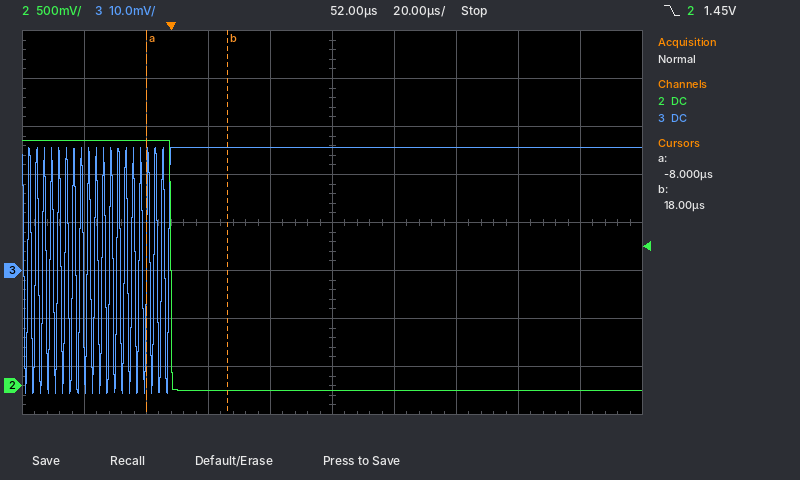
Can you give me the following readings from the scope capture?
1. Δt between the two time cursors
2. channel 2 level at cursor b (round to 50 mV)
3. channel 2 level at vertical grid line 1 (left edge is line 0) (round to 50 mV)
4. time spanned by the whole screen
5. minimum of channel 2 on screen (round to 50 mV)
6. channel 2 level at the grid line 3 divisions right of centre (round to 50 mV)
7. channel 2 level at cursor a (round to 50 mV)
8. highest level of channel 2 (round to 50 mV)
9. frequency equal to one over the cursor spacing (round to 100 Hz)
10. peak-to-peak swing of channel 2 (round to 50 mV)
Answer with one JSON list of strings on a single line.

["26 µs", "-50 mV", "2.55 V", "200 µs", "-50 mV", "-50 mV", "2.55 V", "2.55 V", "38.5 kHz", "2.60 V"]
